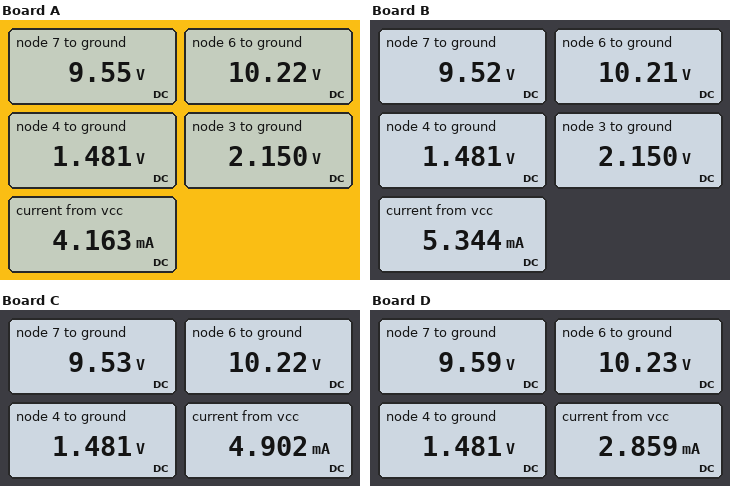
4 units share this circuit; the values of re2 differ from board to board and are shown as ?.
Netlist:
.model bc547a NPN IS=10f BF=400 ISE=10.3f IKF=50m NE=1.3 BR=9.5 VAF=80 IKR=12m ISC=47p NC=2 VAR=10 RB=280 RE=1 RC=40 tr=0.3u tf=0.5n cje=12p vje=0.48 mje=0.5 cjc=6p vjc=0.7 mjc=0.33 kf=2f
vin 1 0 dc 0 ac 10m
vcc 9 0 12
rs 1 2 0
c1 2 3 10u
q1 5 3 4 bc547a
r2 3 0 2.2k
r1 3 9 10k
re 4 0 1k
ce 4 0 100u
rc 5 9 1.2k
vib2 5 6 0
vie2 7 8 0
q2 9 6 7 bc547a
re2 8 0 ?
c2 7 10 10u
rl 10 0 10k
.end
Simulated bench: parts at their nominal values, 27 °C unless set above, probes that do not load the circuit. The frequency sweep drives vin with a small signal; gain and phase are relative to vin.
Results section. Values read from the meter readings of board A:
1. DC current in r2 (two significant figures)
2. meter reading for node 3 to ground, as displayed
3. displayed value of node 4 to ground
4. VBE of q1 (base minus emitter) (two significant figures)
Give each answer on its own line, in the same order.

980 µA
2.150 V
1.481 V
670 mV
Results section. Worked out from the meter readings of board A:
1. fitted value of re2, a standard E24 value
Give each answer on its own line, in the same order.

5.6 kΩ
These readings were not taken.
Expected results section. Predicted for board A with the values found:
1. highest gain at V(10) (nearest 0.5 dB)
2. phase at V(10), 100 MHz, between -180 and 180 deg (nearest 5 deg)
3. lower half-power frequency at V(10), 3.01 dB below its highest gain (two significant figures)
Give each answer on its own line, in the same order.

35.0 dB
20 deg
83 Hz
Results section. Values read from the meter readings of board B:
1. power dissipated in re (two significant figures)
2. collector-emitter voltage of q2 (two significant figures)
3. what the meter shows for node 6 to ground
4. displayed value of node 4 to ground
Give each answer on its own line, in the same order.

2.2 mW
2.5 V
10.21 V
1.481 V
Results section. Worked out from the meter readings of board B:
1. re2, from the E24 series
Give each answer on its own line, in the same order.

3.3 kΩ
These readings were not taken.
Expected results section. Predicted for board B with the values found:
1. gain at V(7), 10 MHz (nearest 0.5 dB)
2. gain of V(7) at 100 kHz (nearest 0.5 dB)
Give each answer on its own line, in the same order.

22.5 dB
35.0 dB
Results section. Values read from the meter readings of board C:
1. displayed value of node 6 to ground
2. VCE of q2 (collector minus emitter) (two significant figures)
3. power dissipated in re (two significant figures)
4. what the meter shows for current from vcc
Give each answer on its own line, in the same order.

10.22 V
2.5 V
2.2 mW
4.902 mA
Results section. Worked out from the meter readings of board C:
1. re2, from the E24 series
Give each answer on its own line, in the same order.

3.9 kΩ
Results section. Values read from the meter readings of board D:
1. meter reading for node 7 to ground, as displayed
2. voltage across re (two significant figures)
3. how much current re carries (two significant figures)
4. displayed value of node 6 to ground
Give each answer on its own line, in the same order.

9.59 V
1.5 V
1.5 mA
10.23 V
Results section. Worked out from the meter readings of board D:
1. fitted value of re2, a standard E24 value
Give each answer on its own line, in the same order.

24 kΩ
